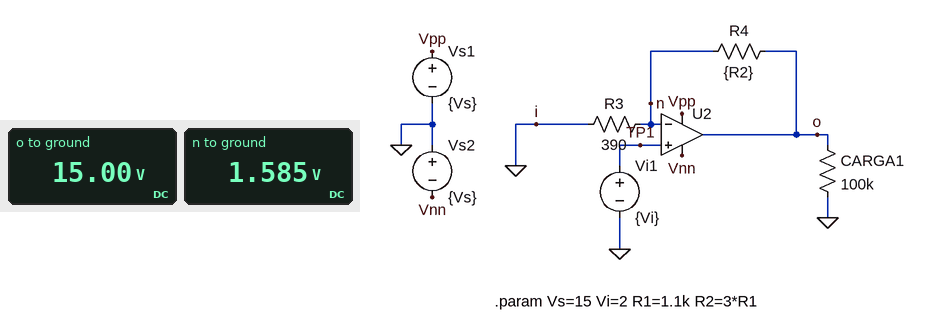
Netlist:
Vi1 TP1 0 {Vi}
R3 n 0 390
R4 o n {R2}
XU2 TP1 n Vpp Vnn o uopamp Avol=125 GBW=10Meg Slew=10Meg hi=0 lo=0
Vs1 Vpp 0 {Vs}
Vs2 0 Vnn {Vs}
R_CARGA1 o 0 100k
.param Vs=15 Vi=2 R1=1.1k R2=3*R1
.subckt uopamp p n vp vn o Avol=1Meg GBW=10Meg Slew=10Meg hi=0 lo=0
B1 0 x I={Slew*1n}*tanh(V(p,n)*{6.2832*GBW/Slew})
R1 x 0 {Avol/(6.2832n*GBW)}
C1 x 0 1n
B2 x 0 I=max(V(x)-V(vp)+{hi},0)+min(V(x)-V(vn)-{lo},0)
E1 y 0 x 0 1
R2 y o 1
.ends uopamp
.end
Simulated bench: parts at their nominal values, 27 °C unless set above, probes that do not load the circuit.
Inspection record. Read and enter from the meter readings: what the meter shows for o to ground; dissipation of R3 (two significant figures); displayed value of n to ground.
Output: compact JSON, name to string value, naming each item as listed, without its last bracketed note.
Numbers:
{"what the meter shows for o to ground": "15.00 V", "dissipation of R3": "6.4 mW", "displayed value of n to ground": "1.585 V"}
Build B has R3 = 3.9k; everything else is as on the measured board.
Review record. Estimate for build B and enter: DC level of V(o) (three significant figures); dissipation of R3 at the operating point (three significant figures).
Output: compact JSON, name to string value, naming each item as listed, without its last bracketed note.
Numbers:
{"DC level of V(o)": "3.64 V", "dissipation of R3 at the operating point": "996 µW"}
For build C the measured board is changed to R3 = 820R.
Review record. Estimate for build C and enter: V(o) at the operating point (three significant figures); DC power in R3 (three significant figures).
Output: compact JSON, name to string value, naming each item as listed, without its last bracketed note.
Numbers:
{"V(o) at the operating point": "9.63 V", "DC power in R3": "4.48 mW"}
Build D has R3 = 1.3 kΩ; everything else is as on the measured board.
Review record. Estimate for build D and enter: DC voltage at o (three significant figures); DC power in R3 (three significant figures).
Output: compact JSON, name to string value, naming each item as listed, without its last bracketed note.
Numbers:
{"DC voltage at o": "6.87 V", "DC power in R3": "2.90 mW"}
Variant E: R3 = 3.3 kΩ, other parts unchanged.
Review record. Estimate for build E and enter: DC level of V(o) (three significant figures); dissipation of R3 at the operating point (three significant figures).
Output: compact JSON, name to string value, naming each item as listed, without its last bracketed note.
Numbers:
{"DC level of V(o)": "3.94 V", "dissipation of R3 at the operating point": "1.17 mW"}
